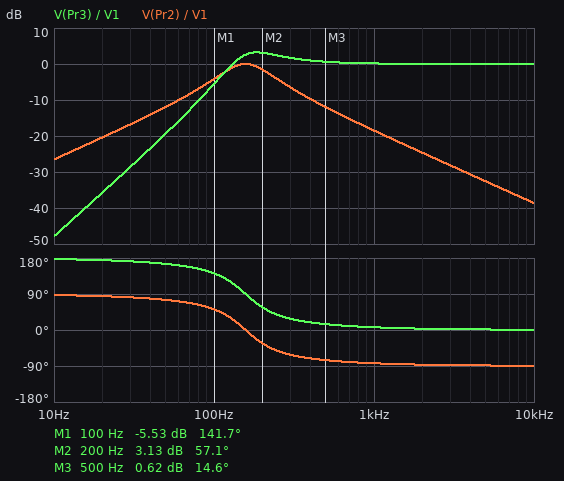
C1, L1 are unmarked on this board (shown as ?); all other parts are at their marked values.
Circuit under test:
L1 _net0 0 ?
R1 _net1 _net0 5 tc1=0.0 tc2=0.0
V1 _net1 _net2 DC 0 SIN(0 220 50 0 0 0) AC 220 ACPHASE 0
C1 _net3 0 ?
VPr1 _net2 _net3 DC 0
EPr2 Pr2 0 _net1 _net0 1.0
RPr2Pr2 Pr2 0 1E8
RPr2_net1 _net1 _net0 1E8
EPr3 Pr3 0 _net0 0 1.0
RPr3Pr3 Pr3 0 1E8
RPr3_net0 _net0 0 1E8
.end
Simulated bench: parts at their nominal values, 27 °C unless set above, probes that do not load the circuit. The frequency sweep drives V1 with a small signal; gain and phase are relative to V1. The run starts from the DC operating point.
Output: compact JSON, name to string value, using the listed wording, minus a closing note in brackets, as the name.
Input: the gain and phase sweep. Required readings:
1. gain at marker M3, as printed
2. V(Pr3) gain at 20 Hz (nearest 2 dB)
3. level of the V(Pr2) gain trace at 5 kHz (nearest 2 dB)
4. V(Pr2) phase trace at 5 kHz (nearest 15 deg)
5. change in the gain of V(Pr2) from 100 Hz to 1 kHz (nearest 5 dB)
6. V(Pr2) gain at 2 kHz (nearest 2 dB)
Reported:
{"gain at marker M3, as printed": "0.62 dB", "V(Pr3) gain at 20 Hz": "-36 dB", "level of the V(Pr2) gain trace at 5 kHz": "-32 dB", "V(Pr2) phase trace at 5 kHz": "-90 deg", "change in the gain of V(Pr2) from 100 Hz to 1 kHz": "-15 dB", "V(Pr2) gain at 2 kHz": "-24 dB"}
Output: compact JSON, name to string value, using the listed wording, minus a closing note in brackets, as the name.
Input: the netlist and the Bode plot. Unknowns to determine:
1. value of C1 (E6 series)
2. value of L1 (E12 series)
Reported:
{"value of C1": "150 µF", "value of L1": "6.8 mH"}
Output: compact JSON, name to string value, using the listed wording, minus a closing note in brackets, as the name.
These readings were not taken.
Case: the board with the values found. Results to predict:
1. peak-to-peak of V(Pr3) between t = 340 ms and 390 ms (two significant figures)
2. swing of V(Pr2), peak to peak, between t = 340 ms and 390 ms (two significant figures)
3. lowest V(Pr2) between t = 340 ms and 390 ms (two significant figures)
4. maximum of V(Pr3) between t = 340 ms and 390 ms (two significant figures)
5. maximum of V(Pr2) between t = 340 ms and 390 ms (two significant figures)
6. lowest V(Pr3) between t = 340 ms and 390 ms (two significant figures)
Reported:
{"peak-to-peak of V(Pr3) between t = 340 ms and 390 ms": "48 V", "swing of V(Pr2), peak to peak, between t = 340 ms and 390 ms": "110 V", "lowest V(Pr2) between t = 340 ms and 390 ms": "-56 V", "maximum of V(Pr3) between t = 340 ms and 390 ms": "24 V", "maximum of V(Pr2) between t = 340 ms and 390 ms": "56 V", "lowest V(Pr3) between t = 340 ms and 390 ms": "-24 V"}
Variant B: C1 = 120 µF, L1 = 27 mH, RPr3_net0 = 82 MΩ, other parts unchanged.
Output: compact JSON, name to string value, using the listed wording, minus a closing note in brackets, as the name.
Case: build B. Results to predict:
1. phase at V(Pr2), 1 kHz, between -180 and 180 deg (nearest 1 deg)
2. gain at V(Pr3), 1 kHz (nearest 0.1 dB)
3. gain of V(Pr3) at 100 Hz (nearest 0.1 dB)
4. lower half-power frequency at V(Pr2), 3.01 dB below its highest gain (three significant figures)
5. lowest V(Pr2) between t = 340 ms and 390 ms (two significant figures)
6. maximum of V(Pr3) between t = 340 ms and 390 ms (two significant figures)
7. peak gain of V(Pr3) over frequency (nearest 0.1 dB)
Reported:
{"phase at V(Pr2), 1 kHz, between -180 and 180 deg": "-88 deg", "gain at V(Pr3), 1 kHz": "0.1 dB", "gain of V(Pr3) at 100 Hz": "8.7 dB", "lower half-power frequency at V(Pr2), 3.01 dB below its highest gain": "74.9 Hz", "lowest V(Pr2) between t = 340 ms and 390 ms": "-59 V", "maximum of V(Pr3) between t = 340 ms and 390 ms": "100 V", "peak gain of V(Pr3) over frequency": "9.7 dB"}
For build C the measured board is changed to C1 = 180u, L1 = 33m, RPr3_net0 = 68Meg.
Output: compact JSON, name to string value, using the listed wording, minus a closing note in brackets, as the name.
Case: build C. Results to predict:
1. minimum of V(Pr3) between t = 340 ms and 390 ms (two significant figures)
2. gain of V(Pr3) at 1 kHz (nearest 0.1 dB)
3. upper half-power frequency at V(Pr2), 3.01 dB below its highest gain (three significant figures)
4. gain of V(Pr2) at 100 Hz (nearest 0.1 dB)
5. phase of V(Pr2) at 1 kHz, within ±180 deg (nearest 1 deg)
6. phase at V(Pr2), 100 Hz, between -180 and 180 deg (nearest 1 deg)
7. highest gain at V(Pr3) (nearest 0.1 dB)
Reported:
{"minimum of V(Pr3) between t = 340 ms and 390 ms": "-260 V", "gain of V(Pr3) at 1 kHz": "0 dB", "upper half-power frequency at V(Pr2), 3.01 dB below its highest gain": "78.5 Hz", "gain of V(Pr2) at 100 Hz": "-8.2 dB", "phase of V(Pr2) at 1 kHz, within ±180 deg": "-89 deg", "phase at V(Pr2), 100 Hz, between -180 and 180 deg": "-67 deg", "highest gain at V(Pr3)": "8.8 dB"}
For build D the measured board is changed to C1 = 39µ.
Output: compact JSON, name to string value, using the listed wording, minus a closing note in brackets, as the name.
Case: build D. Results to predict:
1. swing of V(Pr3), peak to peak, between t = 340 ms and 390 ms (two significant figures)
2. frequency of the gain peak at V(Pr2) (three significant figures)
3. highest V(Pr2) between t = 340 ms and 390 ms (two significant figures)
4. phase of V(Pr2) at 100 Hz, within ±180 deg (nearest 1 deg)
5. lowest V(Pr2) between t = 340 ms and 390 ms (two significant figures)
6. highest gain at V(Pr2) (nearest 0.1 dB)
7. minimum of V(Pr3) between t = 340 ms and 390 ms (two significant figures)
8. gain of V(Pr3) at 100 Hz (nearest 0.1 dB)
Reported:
{"swing of V(Pr3), peak to peak, between t = 340 ms and 390 ms": "12 V", "frequency of the gain peak at V(Pr2)": "309 Hz", "highest V(Pr2) between t = 340 ms and 390 ms": "14 V", "phase of V(Pr2) at 100 Hz, within ±180 deg": "82 deg", "lowest V(Pr2) between t = 340 ms and 390 ms": "-14 V", "highest gain at V(Pr2)": "0 dB", "minimum of V(Pr3) between t = 340 ms and 390 ms": "-5.9 V", "gain of V(Pr3) at 100 Hz": "-18.7 dB"}
